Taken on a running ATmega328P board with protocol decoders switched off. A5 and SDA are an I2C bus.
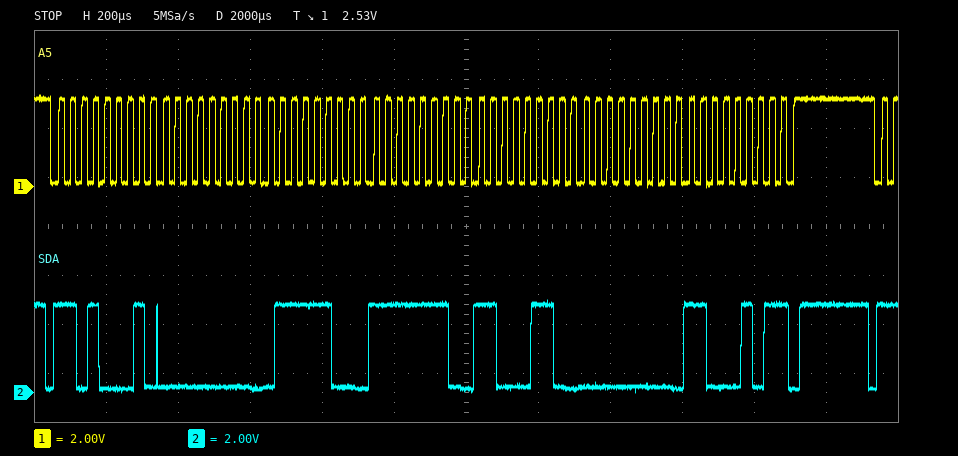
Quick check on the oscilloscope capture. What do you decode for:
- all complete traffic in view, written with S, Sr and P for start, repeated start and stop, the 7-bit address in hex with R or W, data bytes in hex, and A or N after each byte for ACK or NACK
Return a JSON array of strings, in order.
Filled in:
["S 68R A 00 A 7C A FE A C6 A 00 A C5 N P"]
